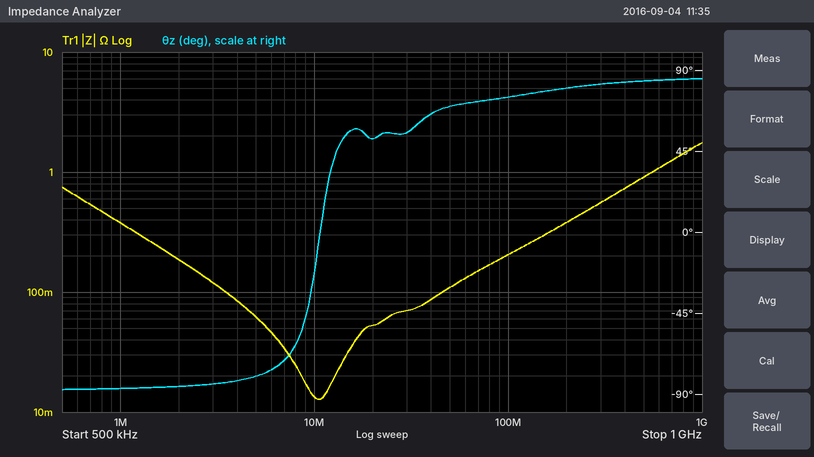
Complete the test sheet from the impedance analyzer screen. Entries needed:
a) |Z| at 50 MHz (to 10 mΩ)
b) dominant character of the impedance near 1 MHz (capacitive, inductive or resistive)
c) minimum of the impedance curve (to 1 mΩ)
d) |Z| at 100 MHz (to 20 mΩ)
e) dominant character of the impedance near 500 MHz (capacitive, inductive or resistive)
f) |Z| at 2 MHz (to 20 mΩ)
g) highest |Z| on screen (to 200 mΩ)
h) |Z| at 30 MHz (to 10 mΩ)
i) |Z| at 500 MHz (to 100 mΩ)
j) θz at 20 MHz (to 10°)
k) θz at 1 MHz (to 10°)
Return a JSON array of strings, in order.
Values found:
["110 mΩ", "capacitive", "13 mΩ", "200 mΩ", "inductive", "180 mΩ", "1.8 Ω", "70 mΩ", "900 mΩ", "50°", "-90°"]
